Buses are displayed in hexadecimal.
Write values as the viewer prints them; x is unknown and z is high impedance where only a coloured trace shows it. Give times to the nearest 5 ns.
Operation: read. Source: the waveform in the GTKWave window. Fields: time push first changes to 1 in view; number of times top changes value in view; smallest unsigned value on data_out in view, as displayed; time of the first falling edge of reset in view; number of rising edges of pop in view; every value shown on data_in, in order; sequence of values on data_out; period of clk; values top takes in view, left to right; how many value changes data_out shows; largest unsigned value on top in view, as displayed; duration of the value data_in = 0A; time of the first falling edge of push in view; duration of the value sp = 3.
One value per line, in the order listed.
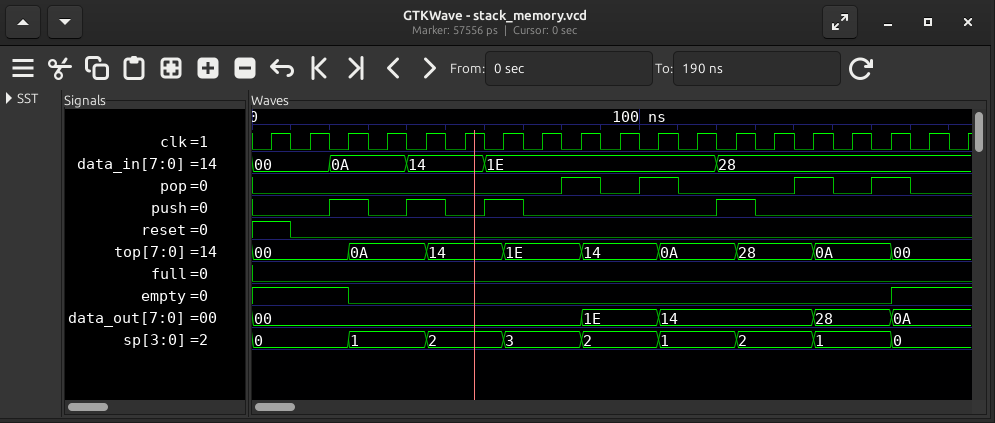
20 ns
8
00
10 ns
4
00, 0A, 14, 1E, 28
00, 1E, 14, 28, 0A
10 ns
00, 0A, 14, 1E, 14, 0A, 28, 0A, 00
4
28
20 ns
30 ns
20 ns
